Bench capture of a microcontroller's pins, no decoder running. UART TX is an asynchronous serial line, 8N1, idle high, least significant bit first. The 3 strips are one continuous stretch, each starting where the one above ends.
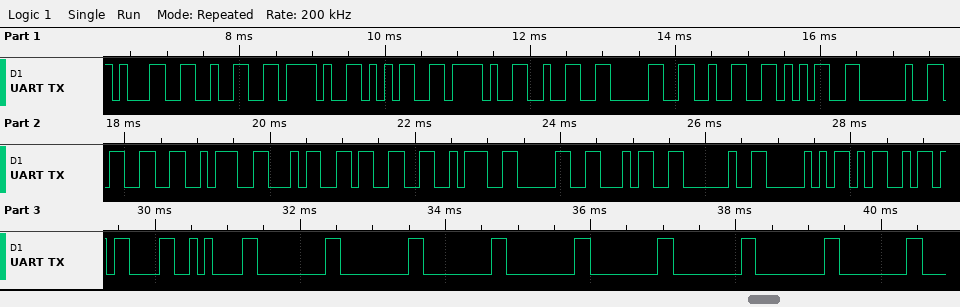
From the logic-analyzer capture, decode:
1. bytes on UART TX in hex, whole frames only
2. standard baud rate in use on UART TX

31 32 2F 35 2F 32 30 32 35 20 33 3A 34 33 3A 30 34 20 50 4D 0D 0A 00 00 00 00 00 00 00 00
9600 baud
